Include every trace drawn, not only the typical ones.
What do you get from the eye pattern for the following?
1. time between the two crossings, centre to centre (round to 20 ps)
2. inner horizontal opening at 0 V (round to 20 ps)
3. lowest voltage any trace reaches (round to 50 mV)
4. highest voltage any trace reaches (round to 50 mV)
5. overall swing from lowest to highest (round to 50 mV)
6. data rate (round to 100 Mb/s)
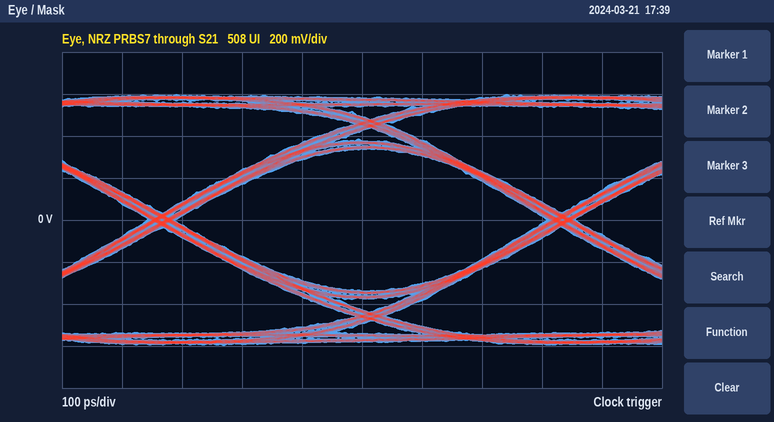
660 ps
620 ps
-600 mV
600 mV
1.20 V
1.5 Gb/s
